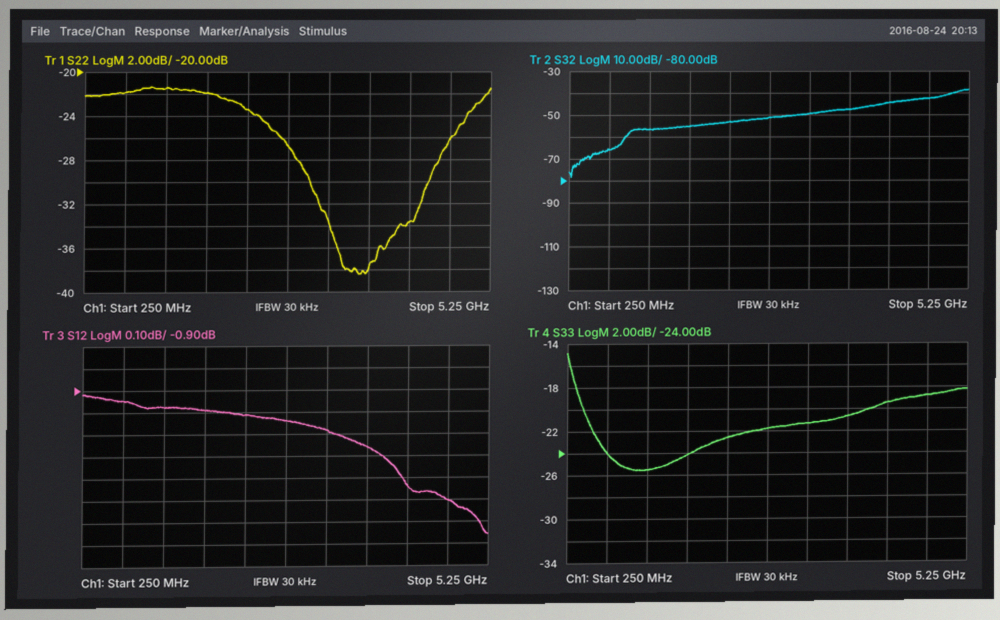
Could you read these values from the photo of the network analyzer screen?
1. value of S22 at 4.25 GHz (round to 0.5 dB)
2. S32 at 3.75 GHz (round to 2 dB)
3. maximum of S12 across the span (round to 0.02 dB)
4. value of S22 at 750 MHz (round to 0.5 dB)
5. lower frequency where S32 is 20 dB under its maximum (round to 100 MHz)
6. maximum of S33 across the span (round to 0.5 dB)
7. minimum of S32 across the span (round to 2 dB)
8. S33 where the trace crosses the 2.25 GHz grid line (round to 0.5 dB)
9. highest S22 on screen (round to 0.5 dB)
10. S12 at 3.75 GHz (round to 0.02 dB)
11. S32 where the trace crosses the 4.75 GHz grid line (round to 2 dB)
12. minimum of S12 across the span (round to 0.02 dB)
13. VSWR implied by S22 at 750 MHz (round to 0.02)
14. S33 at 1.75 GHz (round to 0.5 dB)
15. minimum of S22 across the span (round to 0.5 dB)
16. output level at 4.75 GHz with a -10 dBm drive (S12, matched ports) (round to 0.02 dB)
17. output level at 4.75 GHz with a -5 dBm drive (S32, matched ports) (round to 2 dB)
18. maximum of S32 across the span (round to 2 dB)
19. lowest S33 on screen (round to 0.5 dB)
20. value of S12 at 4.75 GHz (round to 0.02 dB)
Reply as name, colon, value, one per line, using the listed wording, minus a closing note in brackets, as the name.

value of S22 at 4.25 GHz: -33.5 dB
S32 at 3.75 GHz: -48 dB
maximum of S12 across the span: -0.92 dB
value of S22 at 750 MHz: -22.0 dB
lower frequency where S32 is 20 dB under its maximum: 1.0 GHz
maximum of S33 across the span: -15.0 dB
minimum of S32 across the span: -78 dB
S33 where the trace crosses the 2.25 GHz grid line: -22.5 dB
highest S22 on screen: -21.5 dB
S12 at 3.75 GHz: -1.16 dB
S32 where the trace crosses the 4.75 GHz grid line: -42 dB
minimum of S12 across the span: -1.56 dB
VSWR implied by S22 at 750 MHz: 1.18
S33 at 1.75 GHz: -24.0 dB
minimum of S22 across the span: -38.5 dB
output level at 4.75 GHz with a -10 dBm drive (S12, matched ports): -11.40 dBm
output level at 4.75 GHz with a -5 dBm drive (S32, matched ports): -48 dBm
maximum of S32 across the span: -38 dB
lowest S33 on screen: -25.5 dB
value of S12 at 4.75 GHz: -1.40 dB
